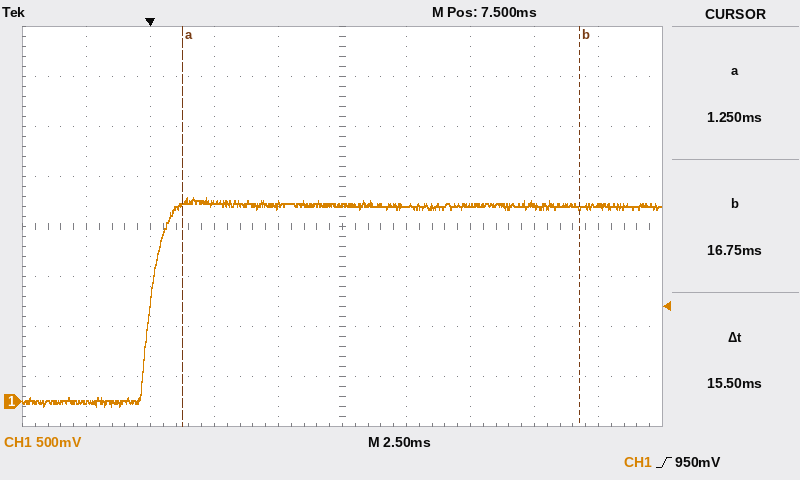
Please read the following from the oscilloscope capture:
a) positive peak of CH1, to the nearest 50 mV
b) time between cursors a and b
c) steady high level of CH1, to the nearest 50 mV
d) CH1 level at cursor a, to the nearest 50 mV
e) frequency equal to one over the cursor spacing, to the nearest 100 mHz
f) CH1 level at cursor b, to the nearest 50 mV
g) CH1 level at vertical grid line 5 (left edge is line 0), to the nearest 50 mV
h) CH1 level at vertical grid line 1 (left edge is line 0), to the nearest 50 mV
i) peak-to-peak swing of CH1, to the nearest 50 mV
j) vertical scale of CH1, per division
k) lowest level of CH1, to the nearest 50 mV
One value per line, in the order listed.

2.05 V
15.5 ms
1.95 V
2.00 V
64.5 Hz
1.95 V
1.95 V
0 mV
2.10 V
500 mV
-50 mV
